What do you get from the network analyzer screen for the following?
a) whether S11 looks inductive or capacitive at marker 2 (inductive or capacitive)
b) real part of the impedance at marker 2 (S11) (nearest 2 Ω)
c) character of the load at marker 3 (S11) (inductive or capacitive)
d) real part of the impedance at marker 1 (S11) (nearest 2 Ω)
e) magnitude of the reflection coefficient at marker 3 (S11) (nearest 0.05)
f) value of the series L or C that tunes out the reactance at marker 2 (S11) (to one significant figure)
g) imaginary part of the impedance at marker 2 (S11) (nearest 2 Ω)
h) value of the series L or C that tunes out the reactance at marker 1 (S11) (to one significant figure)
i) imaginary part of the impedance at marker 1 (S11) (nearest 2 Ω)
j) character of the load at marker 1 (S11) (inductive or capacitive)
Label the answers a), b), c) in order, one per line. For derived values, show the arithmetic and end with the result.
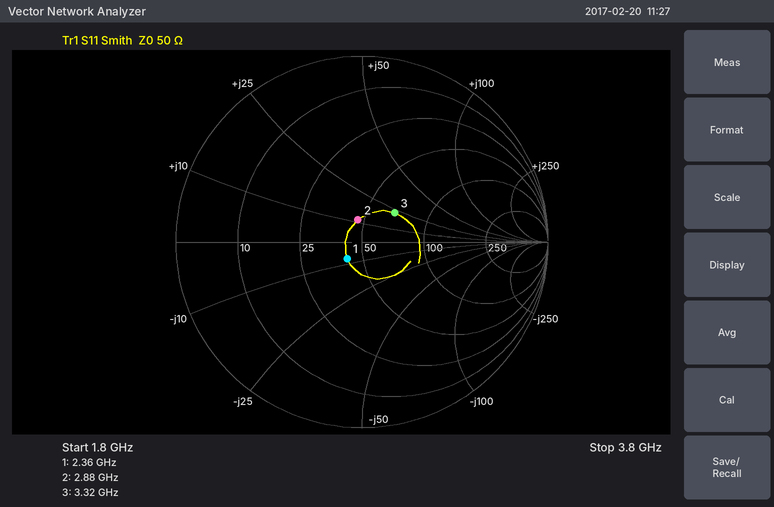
a) inductive
b) 46 Ω
c) inductive
d) 42 Ω
e) 0.25
f) C = 1/(2π × 2.88 GHz × 12 Ω) ≈ 5 pF
g) +12 Ω
h) L = 8 Ω/(2π × 2.36 GHz) ≈ 540 pH, so 500 pH to one significant figure
i) -8 Ω
j) capacitive
